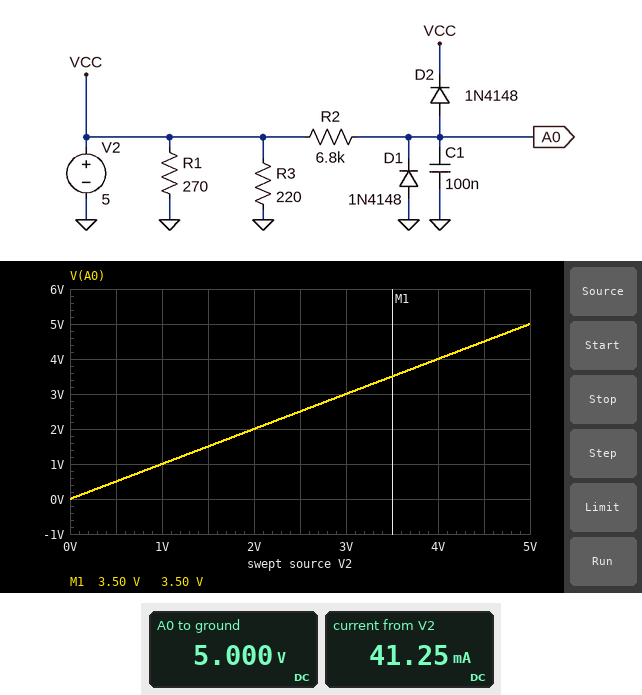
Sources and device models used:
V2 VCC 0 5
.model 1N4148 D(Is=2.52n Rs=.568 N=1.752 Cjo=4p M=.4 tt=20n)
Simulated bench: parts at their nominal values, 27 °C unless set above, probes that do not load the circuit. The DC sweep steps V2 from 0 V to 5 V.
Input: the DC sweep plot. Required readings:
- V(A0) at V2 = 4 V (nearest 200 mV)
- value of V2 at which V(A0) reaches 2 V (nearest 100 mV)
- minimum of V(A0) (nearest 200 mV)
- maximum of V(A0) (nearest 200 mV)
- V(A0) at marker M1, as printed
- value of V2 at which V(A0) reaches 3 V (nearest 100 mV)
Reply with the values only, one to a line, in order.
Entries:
4.0 V
2.0 V
0 V
5.0 V
3.50 V
3.0 V
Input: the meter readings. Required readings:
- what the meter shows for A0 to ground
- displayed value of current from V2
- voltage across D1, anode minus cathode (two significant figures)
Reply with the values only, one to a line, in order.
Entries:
5.000 V
41.25 mA
-5.0 V
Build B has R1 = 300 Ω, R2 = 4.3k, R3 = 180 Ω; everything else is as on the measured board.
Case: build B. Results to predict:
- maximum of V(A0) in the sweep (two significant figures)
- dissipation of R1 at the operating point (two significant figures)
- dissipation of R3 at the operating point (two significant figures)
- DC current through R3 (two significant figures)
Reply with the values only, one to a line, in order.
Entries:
5.0 V
83 mW
140 mW
28 mA
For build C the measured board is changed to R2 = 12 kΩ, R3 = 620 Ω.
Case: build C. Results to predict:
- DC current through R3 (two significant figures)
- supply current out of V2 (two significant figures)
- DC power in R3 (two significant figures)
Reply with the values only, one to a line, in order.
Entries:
8.1 mA
27 mA
40 mW
